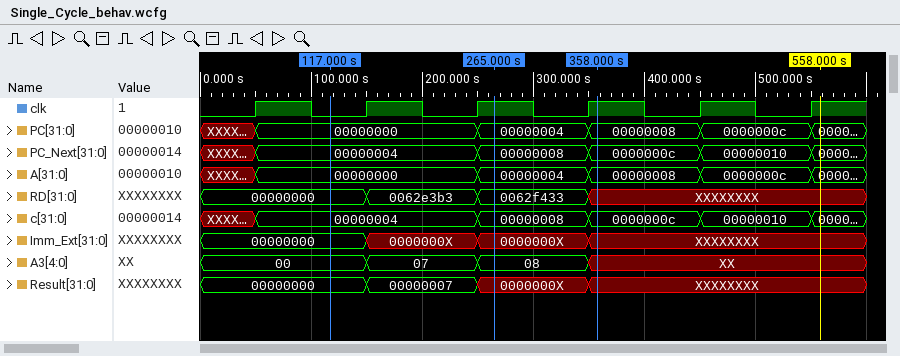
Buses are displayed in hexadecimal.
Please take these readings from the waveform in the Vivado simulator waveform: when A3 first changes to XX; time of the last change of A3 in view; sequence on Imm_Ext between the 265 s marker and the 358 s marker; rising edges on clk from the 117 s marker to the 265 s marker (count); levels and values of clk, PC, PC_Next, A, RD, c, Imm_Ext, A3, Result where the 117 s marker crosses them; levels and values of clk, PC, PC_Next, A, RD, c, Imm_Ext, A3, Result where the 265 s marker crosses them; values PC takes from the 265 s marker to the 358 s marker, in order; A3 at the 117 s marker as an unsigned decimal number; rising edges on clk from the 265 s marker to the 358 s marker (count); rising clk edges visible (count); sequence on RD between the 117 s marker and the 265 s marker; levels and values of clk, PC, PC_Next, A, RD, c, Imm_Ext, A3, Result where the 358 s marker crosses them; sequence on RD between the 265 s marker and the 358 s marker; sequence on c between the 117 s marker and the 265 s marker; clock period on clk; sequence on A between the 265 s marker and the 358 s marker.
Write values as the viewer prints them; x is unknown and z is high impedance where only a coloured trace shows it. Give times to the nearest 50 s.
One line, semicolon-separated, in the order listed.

350 s; 350 s; 0000000X, XXXXXXXX; 2; clk=0, PC=00000000, PC_Next=00000004, A=00000000, RD=00000000, c=00000004, Imm_Ext=00000000, A3=00, Result=00000000; clk=1, PC=00000004, PC_Next=00000008, A=00000004, RD=0062f433, c=00000008, Imm_Ext=0000000X, A3=08, Result=0000000X; 00000004, 00000008; 0; 1; 6; 00000000, 0062e3b3, 0062f433; clk=1, PC=00000008, PC_Next=0000000c, A=00000008, RD=XXXXXXXX, c=0000000c, Imm_Ext=XXXXXXXX, A3=XX, Result=XXXXXXXX; 0062f433, XXXXXXXX; 00000004, 00000008; 100 s; 00000004, 00000008
